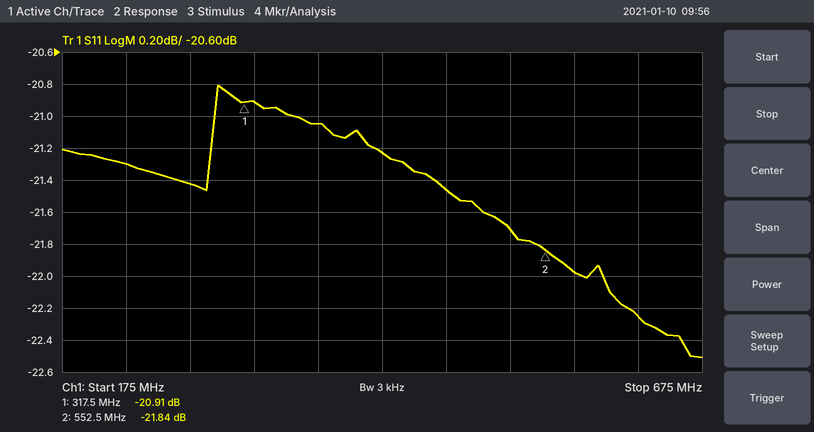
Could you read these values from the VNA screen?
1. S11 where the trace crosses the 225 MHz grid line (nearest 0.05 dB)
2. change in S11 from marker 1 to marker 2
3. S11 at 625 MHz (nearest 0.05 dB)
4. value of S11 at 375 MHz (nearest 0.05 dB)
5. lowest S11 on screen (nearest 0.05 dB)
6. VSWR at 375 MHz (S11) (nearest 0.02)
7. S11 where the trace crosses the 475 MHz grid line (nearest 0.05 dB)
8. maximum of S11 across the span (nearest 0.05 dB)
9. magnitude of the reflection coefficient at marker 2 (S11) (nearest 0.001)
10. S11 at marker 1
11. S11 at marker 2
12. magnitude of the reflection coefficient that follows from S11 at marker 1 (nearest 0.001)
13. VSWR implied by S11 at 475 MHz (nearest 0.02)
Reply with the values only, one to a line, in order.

-21.30 dB
-0.93 dB
-22.25 dB
-21.05 dB
-22.50 dB
1.20
-21.45 dB
-20.80 dB
0.081
-20.91 dB
-21.84 dB
0.090
1.18
